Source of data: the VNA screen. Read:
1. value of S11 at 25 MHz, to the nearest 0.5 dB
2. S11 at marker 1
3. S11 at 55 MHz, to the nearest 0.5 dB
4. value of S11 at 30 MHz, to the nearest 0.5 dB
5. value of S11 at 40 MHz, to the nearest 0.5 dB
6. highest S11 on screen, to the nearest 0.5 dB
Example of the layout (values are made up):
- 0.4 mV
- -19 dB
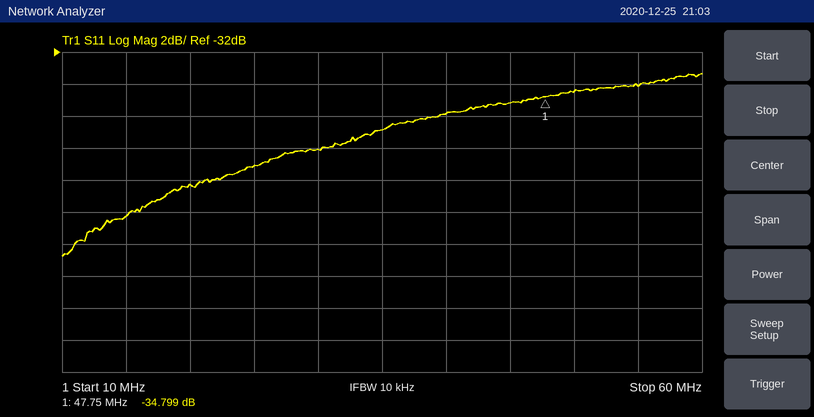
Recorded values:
- -39.0 dB
- -34.799 dB
- -34.0 dB
- -38.0 dB
- -36.0 dB
- -33.5 dB
